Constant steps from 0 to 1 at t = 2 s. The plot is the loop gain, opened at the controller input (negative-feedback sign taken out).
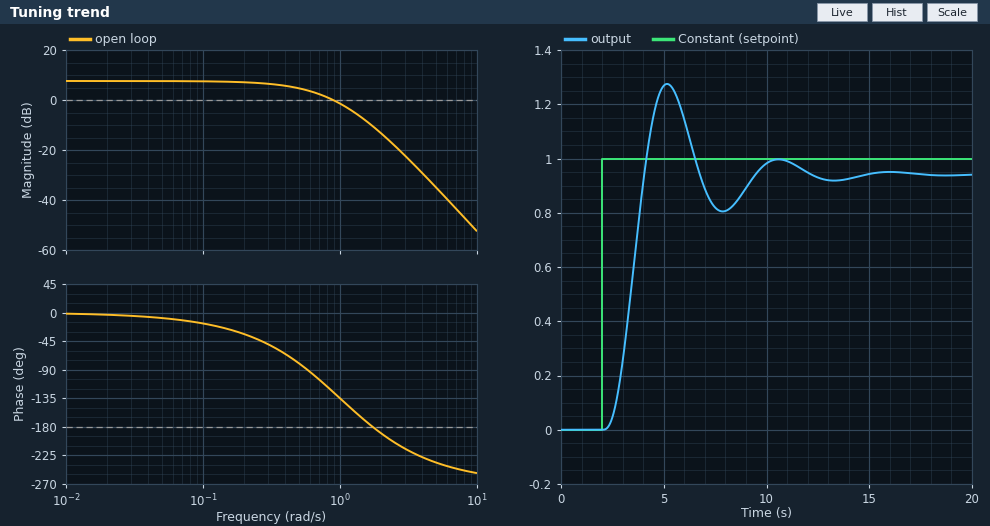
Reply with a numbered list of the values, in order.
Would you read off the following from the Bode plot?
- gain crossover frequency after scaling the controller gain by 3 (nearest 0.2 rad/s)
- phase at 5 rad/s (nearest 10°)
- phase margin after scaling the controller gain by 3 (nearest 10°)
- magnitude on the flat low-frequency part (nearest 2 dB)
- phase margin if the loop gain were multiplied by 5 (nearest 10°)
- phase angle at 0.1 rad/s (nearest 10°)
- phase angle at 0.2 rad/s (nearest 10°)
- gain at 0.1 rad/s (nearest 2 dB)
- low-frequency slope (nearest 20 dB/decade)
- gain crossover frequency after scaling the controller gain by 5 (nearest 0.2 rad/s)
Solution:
1. 1.6 rad/s
2. -240°
3. 0°
4. 8 dB
5. -10°
6. -20°
7. -30°
8. 8 dB
9. 0 dB/decade
10. 2.0 rad/s
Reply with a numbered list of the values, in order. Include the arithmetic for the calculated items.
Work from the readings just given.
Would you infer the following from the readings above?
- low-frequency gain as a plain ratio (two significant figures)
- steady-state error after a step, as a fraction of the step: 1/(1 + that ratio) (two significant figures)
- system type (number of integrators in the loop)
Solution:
1. 10^(8 / 20) = 2.5
2. 1 / (1 + 2.5) = 0.29
3. 0
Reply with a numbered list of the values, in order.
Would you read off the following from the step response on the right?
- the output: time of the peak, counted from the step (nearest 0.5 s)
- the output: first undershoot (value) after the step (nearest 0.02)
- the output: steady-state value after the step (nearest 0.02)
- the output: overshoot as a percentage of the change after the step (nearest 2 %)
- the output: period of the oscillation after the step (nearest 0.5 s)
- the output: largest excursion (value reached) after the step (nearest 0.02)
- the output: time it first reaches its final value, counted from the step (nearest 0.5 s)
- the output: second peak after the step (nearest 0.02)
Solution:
1. 3.0 s
2. 0.80
3. 0.94
4. 36 %
5. 5.5 s
6. 1.28
7. 2.0 s
8. 1.00
